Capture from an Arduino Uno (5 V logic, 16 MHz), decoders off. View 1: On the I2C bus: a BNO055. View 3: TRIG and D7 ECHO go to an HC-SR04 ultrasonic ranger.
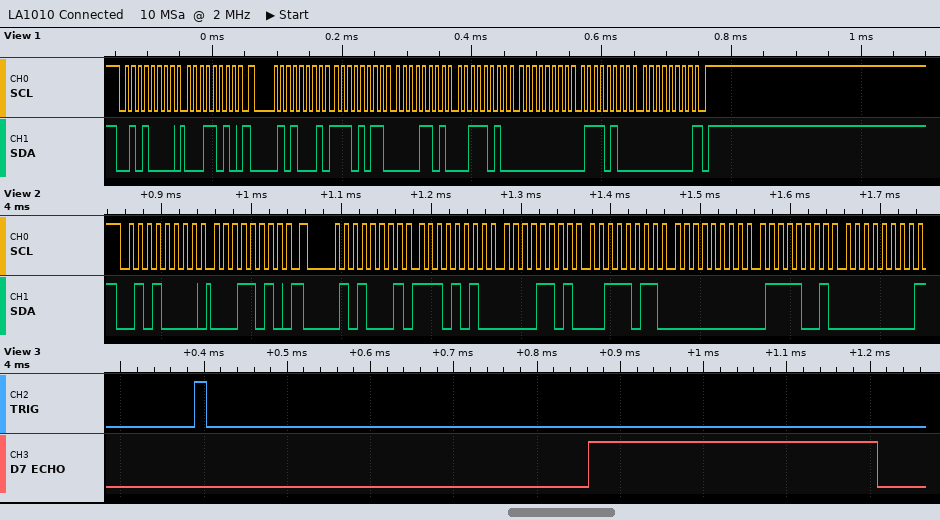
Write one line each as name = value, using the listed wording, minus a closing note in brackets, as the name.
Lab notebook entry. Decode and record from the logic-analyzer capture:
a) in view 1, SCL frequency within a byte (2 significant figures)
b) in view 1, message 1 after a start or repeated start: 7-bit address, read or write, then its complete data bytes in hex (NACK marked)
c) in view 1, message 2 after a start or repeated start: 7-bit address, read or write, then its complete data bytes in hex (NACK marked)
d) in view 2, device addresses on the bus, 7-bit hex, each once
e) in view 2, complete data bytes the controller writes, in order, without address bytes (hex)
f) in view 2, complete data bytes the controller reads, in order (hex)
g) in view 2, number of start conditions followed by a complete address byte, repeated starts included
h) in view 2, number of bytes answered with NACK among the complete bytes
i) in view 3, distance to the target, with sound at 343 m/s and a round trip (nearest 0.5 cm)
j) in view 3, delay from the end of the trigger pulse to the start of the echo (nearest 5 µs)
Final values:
in view 1, SCL frequency within a byte = 100 kHz
in view 1, message 1 after a start or repeated start: 7-bit address, read or write, then its complete data bytes in hex = 0x28 write: 1A
in view 1, message 2 after a start or repeated start: 7-bit address, read or write, then its complete data bytes in hex = 0x28 read: EB 0D 3A 00 74 00 NACK
in view 2, device addresses on the bus, 7-bit hex, each once = 0x28
in view 2, complete data bytes the controller writes, in order, without address bytes = 1A
in view 2, complete data bytes the controller reads, in order = EA 0D 3B 00 79 00
in view 2, number of start conditions followed by a complete address byte, repeated starts included = 2
in view 2, number of bytes answered with NACK among the complete bytes = 1
in view 3, distance to the target, with sound at 343 m/s and a round trip = 6 cm
in view 3, delay from the end of the trigger pulse to the start of the echo = 460 µs
